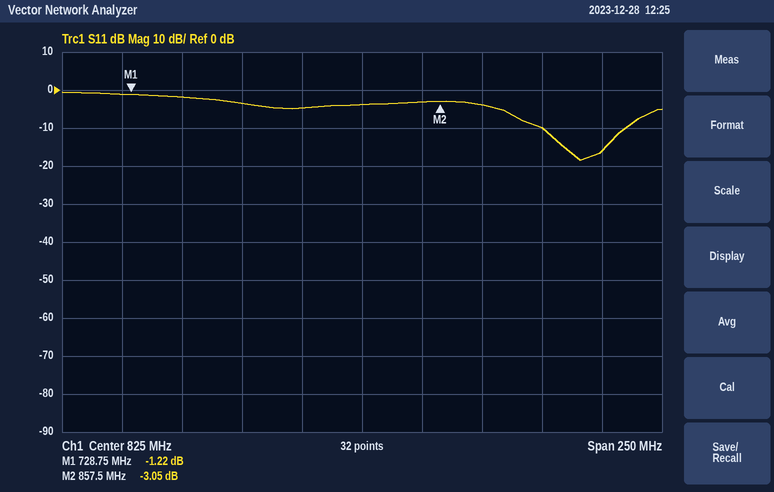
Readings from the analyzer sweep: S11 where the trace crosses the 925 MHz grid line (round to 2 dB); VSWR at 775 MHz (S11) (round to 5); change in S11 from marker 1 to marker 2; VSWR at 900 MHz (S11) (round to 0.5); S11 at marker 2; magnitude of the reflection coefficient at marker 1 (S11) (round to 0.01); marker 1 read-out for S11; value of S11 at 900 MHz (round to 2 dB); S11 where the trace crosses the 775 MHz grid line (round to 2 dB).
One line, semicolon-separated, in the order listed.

-16 dB; 5; -1.83 dB; 2.0; -3.05 dB; 0.87; -1.22 dB; -10 dB; -4 dB
